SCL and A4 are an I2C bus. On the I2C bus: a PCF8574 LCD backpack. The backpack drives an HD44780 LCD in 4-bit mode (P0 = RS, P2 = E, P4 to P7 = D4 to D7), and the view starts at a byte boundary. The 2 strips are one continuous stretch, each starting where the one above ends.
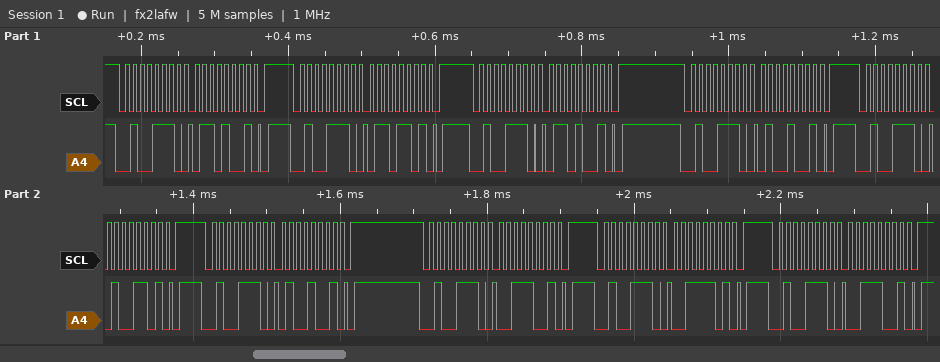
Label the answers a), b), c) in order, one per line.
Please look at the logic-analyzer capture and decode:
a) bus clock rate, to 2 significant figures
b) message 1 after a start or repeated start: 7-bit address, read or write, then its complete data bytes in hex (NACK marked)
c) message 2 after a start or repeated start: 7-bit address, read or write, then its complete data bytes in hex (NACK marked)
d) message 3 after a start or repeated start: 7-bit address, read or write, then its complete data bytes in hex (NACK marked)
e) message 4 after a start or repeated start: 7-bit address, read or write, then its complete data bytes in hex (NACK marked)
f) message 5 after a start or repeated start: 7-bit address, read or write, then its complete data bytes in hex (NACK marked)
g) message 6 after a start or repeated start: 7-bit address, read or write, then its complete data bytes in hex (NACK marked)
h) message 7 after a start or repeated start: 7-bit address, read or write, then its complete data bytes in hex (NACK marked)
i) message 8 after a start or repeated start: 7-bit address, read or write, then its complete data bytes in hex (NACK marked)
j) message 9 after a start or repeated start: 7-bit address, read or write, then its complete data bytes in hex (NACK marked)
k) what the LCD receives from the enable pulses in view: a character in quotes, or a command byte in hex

a) 100 kHz
b) 0x27 write: 69
c) 0x27 write: 6D
d) 0x27 write: 69
e) 0x27 write: 49
f) 0x27 write: 4D
g) 0x27 write: 49
h) 0x27 write: 39
i) 0x27 write: 3D
j) 0x27 write: 39
k) 'd'
